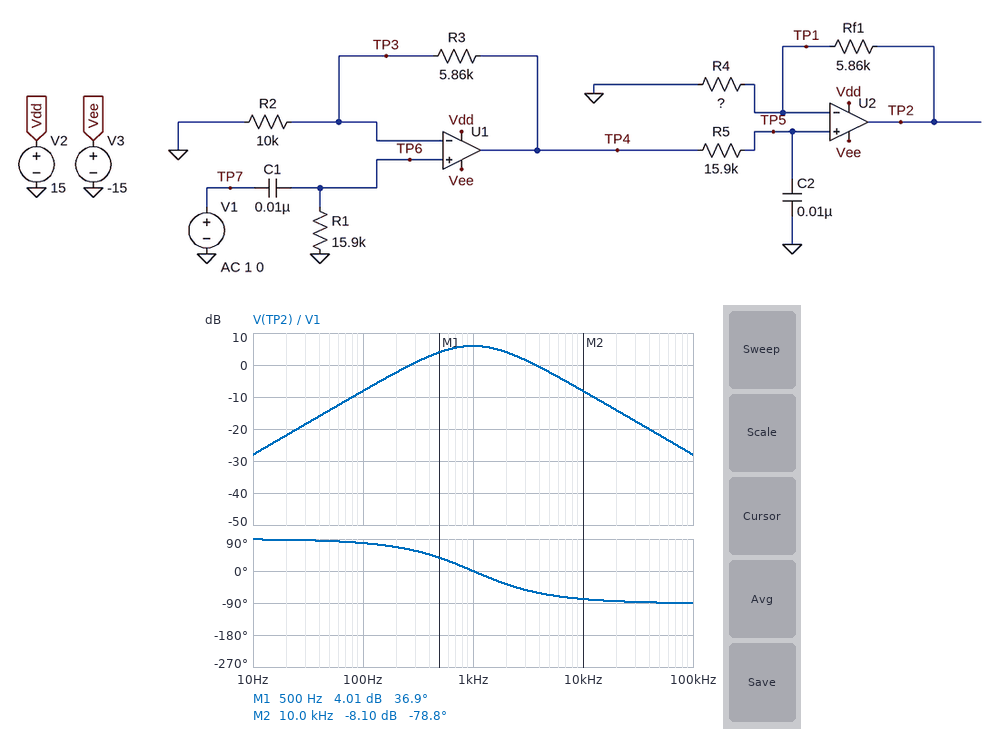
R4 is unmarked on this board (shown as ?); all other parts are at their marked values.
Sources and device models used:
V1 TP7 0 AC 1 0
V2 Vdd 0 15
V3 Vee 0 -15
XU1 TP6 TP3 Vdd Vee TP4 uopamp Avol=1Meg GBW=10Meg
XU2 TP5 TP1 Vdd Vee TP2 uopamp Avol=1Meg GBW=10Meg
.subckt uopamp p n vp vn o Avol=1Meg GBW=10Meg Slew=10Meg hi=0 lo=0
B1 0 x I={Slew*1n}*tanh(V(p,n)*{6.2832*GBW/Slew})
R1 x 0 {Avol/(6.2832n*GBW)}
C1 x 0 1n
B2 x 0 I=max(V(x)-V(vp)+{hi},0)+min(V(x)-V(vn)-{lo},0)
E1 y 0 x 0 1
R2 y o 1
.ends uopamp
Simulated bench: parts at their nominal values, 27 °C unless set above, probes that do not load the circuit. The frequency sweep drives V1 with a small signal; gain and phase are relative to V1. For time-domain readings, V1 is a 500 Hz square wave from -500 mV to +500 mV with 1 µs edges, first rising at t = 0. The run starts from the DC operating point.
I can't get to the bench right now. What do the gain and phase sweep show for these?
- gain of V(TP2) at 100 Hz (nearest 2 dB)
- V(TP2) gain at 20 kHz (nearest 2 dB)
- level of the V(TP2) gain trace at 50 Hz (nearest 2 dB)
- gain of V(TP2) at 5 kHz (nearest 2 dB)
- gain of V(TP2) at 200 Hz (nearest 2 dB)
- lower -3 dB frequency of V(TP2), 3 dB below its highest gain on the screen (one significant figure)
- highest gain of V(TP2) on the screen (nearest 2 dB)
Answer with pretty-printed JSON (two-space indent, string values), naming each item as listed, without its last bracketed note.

{
  "gain of V(TP2) at 100 Hz": "-8 dB",
  "V(TP2) gain at 20 kHz": "-14 dB",
  "level of the V(TP2) gain trace at 50 Hz": "-14 dB",
  "gain of V(TP2) at 5 kHz": "-2 dB",
  "gain of V(TP2) at 200 Hz": "-2 dB",
  "lower -3 dB frequency of V(TP2), 3 dB below its highest gain on the screen": "400 Hz",
  "highest gain of V(TP2) on the screen": "6 dB"
}
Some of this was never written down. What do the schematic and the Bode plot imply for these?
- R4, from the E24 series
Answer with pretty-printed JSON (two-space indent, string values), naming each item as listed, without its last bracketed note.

{
  "R4, from the E24 series": "3.9 kΩ"
}
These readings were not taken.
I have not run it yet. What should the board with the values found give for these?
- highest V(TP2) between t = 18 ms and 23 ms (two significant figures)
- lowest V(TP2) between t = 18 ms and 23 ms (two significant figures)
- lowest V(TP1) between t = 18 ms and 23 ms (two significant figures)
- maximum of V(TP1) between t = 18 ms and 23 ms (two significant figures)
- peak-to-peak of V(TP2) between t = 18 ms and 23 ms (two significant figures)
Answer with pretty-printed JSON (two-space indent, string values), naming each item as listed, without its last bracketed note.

{
  "highest V(TP2) between t = 18 ms and 23 ms": "1.4 V",
  "lowest V(TP2) between t = 18 ms and 23 ms": "-1.4 V",
  "lowest V(TP1) between t = 18 ms and 23 ms": "-580 mV",
  "maximum of V(TP1) between t = 18 ms and 23 ms": "580 mV",
  "peak-to-peak of V(TP2) between t = 18 ms and 23 ms": "2.9 V"
}
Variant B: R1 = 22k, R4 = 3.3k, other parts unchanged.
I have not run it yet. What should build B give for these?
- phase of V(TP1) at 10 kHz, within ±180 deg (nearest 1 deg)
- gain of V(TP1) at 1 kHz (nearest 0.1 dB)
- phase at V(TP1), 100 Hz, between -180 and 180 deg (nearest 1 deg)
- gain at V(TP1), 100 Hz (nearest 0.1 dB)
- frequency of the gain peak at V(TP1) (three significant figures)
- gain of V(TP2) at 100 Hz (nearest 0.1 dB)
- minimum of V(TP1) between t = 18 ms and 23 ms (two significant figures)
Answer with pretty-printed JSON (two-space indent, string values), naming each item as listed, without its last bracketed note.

{
  "phase of V(TP1) at 10 kHz, within ±180 deg": "-80 deg",
  "gain of V(TP1) at 1 kHz": "-0.8 dB",
  "phase at V(TP1), 100 Hz, between -180 and 180 deg": "76 deg",
  "gain at V(TP1), 100 Hz": "-13.3 dB",
  "frequency of the gain peak at V(TP1)": "851 Hz",
  "gain of V(TP2) at 100 Hz": "-4.4 dB",
  "minimum of V(TP1) between t = 18 ms and 23 ms": "-660 mV"
}
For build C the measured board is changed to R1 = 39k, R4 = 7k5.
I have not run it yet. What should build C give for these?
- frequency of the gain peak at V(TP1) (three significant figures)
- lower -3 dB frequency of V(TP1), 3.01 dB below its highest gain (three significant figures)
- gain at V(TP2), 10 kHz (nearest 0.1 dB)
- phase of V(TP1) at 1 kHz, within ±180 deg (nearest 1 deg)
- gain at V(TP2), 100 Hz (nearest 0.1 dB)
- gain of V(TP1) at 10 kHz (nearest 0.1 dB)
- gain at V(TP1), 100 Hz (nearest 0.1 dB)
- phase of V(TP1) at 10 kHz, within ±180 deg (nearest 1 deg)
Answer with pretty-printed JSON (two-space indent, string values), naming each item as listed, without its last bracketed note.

{
  "frequency of the gain peak at V(TP1)": "639 Hz",
  "lower -3 dB frequency of V(TP1), 3.01 dB below its highest gain": "247 Hz",
  "gain at V(TP2), 10 kHz": "-11.0 dB",
  "phase of V(TP1) at 1 kHz, within ±180 deg": "-23 deg",
  "gain at V(TP2), 100 Hz": "-3.5 dB",
  "gain of V(TP1) at 10 kHz": "-16.0 dB",
  "gain at V(TP1), 100 Hz": "-8.5 dB",
  "phase of V(TP1) at 10 kHz, within ±180 deg": "-82 deg"
}
